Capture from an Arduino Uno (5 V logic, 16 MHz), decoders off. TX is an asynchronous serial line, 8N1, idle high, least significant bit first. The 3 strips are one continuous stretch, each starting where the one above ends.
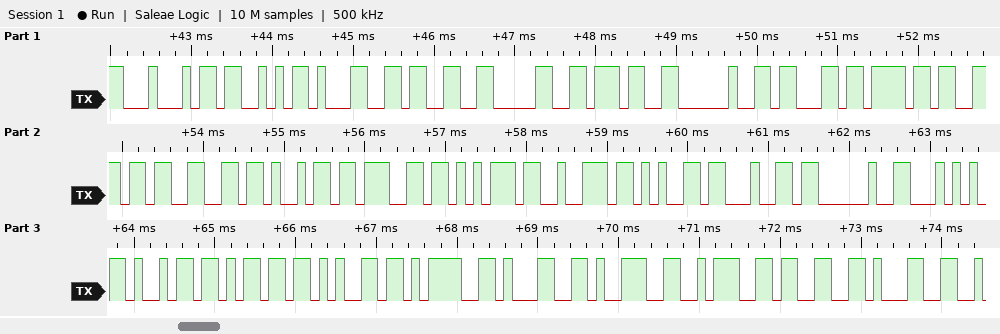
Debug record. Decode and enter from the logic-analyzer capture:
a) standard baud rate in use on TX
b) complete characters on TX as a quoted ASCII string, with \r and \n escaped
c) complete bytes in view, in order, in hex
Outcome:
9600 baud
"DS1307 configured Time=19:31"
44 53 31 33 30 37 20 63 6F 6E 66 69 67 75 72 65 64 20 54 69 6D 65 3D 31 39 3A 33 31
